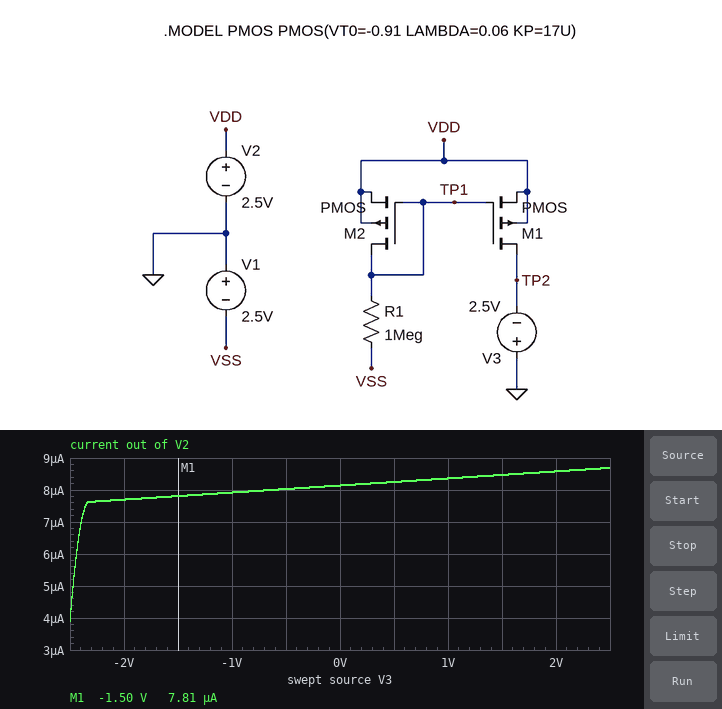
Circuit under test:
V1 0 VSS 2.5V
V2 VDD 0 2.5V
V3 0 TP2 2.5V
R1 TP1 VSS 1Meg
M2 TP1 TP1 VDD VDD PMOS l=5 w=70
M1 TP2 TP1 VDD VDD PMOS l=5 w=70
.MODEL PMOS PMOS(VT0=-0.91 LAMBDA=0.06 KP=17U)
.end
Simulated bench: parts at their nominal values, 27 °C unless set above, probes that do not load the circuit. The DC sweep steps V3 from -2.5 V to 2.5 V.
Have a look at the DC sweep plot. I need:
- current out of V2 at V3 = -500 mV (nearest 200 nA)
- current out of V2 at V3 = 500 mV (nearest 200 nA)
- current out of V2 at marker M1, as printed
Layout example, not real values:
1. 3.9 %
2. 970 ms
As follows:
1. 8.0 µA
2. 8.2 µA
3. 7.81 µA
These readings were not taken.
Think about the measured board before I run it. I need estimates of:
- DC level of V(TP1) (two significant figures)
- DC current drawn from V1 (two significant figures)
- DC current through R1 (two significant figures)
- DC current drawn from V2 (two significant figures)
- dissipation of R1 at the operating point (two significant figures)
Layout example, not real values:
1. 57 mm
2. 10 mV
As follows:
1. 1.4 V
2. 3.9 µA
3. 3.9 µA
4. 8.7 µA
5. 15 µW
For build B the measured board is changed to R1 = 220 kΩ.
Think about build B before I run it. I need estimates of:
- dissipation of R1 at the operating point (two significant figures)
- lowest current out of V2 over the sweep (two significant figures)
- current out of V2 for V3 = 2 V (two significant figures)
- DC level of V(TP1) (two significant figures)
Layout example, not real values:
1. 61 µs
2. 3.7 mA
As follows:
1. 63 µW
2. 17 µA
3. 37 µA
4. 1.2 V
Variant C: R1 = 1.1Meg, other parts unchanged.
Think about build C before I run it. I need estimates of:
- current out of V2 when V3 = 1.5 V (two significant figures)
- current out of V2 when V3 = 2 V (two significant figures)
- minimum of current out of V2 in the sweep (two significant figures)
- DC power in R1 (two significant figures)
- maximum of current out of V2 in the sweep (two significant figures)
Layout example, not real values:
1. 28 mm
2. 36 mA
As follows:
1. 7.7 µA
2. 7.8 µA
3. 3.6 µA
4. 14 µW
5. 7.9 µA
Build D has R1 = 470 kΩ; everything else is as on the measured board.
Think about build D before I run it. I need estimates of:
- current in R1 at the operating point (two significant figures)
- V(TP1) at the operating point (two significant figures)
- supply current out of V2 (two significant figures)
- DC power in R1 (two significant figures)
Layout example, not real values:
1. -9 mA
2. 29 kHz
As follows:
1. 8.2 µA
2. 1.3 V
3. 18 µA
4. 31 µW
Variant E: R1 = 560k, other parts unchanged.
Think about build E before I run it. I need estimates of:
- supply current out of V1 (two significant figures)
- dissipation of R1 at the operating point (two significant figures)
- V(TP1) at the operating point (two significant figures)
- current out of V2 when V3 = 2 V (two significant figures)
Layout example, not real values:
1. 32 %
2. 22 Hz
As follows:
1. 6.9 µA
2. 27 µW
3. 1.4 V
4. 15 µA
